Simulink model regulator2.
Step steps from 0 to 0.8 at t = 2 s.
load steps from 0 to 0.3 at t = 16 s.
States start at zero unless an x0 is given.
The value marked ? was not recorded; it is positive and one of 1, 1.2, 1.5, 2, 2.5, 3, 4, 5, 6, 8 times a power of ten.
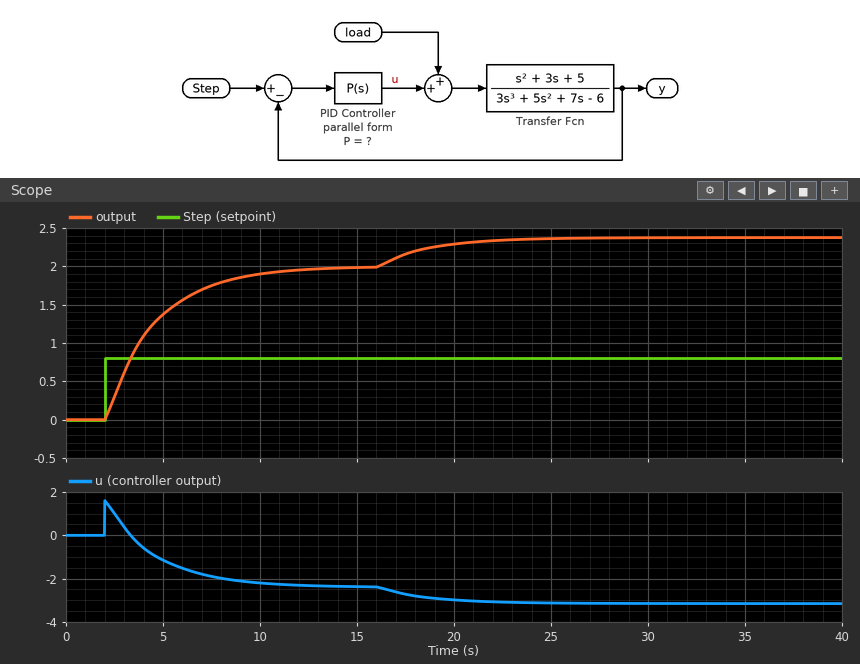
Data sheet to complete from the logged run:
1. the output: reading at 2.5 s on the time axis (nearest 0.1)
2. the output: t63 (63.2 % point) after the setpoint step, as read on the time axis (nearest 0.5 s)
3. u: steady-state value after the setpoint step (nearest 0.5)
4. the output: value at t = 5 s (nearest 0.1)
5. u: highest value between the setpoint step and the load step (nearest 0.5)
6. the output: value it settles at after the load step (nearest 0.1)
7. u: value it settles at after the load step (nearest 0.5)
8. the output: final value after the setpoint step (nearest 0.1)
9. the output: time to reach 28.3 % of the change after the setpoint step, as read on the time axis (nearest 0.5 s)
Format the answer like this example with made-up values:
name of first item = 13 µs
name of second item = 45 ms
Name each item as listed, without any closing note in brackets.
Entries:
the output: reading at 2.5 s on the time axis = 0.3
the output: t63 (63.2 % point) after the setpoint step, as read on the time axis = 4.5 s
u: steady-state value after the setpoint step = -2.5
the output: value at t = 5 s = 1.4
u: highest value between the setpoint step and the load step = 1.5
the output: value it settles at after the load step = 2.4
u: value it settles at after the load step = -3.0
the output: final value after the setpoint step = 2.0
the output: time to reach 28.3 % of the change after the setpoint step, as read on the time axis = 3.0 s
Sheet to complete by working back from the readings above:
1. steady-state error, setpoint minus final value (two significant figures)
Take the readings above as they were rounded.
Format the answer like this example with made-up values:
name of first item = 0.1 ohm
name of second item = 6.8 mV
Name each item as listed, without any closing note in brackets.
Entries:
steady-state error, setpoint minus final value = -1.2
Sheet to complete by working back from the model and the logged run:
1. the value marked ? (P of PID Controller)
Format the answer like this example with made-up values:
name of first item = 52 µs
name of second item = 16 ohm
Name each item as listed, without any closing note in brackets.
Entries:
the value marked ? = 2
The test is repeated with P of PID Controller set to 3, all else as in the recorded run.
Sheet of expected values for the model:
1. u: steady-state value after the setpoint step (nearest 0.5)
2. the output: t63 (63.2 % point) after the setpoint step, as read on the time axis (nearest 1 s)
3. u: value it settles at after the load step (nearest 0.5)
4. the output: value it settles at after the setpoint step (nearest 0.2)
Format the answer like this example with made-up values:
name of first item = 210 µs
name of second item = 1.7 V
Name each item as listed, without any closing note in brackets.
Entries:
u: steady-state value after the setpoint step = -1.5
the output: t63 (63.2 % point) after the setpoint step, as read on the time axis = 3 s
u: value it settles at after the load step = -2.0
the output: value it settles at after the setpoint step = 1.4
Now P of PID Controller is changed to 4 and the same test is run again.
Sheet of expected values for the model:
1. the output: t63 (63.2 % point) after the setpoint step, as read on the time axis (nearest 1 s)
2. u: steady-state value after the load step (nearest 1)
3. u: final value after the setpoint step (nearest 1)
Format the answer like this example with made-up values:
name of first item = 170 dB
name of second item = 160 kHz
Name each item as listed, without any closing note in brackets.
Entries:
the output: t63 (63.2 % point) after the setpoint step, as read on the time axis = 3 s
u: steady-state value after the load step = -2
u: final value after the setpoint step = -1
